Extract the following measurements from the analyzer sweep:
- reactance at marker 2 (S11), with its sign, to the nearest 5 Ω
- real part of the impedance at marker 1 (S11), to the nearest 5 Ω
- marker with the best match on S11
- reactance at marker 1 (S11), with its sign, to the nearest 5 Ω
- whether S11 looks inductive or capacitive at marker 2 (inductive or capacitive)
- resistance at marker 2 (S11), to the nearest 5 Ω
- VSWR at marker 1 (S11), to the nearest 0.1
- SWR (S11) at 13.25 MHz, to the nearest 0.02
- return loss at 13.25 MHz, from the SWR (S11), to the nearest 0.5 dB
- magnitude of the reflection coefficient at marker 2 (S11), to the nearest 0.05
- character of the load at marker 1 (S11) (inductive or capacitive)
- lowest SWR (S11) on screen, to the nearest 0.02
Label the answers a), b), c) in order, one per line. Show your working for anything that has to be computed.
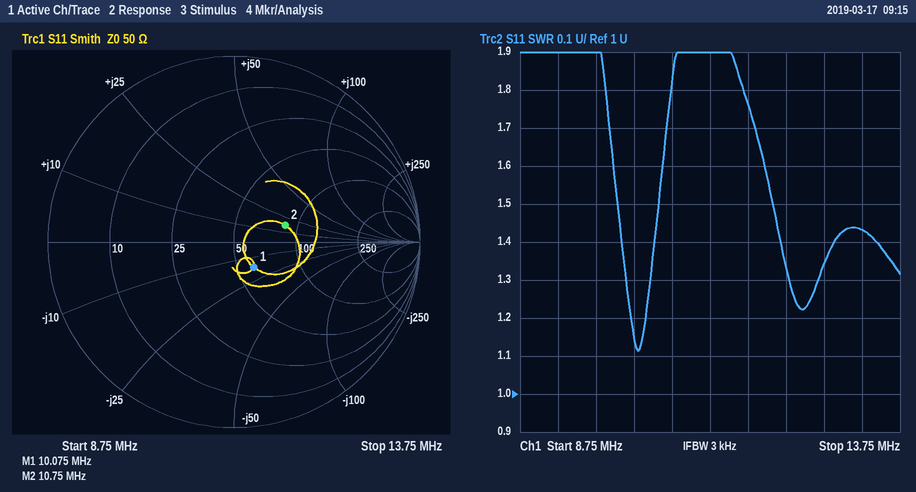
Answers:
a) +15 Ω
b) 60 Ω
c) marker 1
d) -15 Ω
e) inductive
f) 85 Ω
g) 1.4
h) 1.44
i) −20 log10((1.44 − 1)/(1.44 + 1)) ≈ 14.9 dB, so 15.0 dB to the nearest 0.5 dB
j) 0.30
k) capacitive
l) 1.12
